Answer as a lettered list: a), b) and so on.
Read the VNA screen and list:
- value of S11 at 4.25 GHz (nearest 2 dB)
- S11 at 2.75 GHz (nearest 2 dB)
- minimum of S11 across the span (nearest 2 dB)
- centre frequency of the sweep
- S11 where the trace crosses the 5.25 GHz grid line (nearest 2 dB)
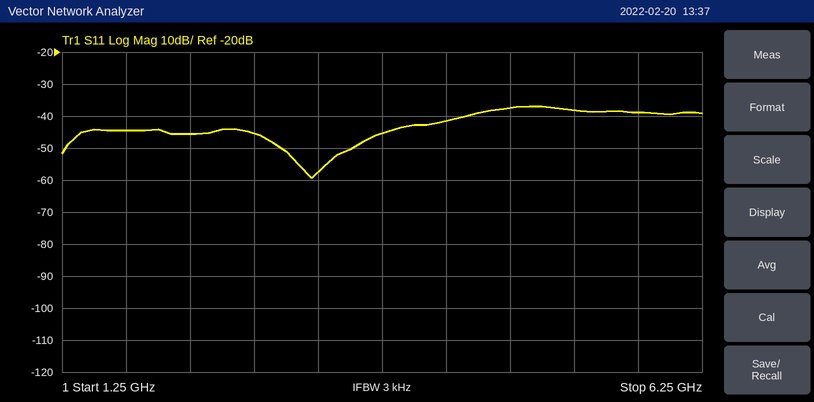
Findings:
a) -42 dB
b) -46 dB
c) -60 dB
d) 3.75 GHz
e) -38 dB
